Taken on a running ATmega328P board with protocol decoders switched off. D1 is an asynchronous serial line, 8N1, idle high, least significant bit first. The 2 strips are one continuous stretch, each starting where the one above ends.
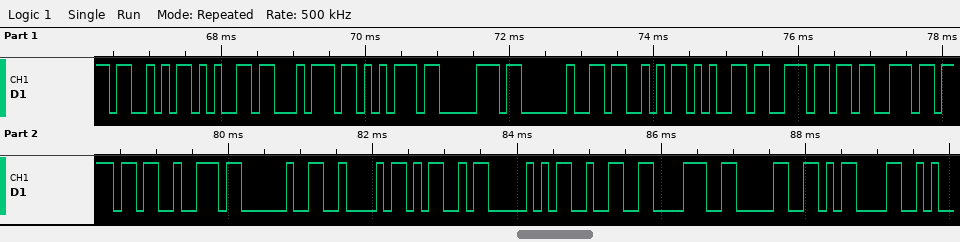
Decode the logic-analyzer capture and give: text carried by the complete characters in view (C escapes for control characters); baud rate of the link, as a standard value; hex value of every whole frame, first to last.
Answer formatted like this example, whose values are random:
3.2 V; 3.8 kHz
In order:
"Setup Sensor BMP280\r"; 9600 baud; 53 65 74 75 70 20 53 65 6E 73 6F 72 20 42 4D 50 32 38 30 0D
